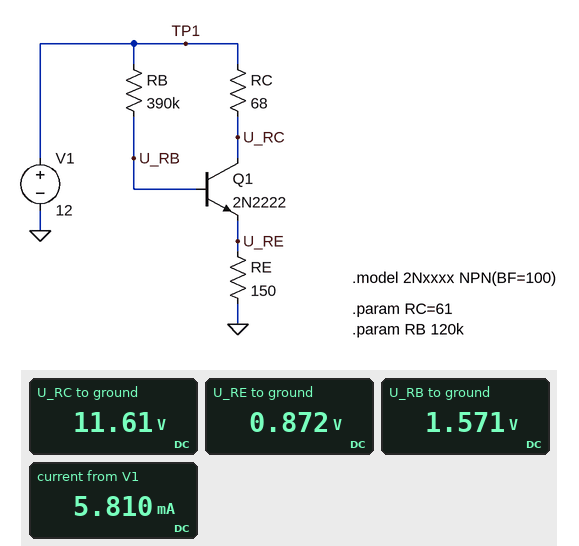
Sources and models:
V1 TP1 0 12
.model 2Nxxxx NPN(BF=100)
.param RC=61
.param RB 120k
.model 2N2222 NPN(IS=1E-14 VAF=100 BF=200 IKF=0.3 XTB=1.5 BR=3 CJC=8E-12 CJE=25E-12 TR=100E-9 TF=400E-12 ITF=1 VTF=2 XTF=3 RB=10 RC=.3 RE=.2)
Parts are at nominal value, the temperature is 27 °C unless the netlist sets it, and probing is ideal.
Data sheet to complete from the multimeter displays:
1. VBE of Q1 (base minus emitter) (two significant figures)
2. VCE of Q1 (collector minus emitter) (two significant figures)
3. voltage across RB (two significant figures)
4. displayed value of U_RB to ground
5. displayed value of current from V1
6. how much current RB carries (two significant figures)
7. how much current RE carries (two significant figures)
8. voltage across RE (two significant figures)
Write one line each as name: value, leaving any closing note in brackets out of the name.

VBE of Q1 (base minus emitter): 700 mV
VCE of Q1 (collector minus emitter): 11 V
voltage across RB: 10 V
displayed value of U_RB to ground: 1.571 V
displayed value of current from V1: 5.810 mA
how much current RB carries: 27 µA
how much current RE carries: 5.8 mA
voltage across RE: 870 mV
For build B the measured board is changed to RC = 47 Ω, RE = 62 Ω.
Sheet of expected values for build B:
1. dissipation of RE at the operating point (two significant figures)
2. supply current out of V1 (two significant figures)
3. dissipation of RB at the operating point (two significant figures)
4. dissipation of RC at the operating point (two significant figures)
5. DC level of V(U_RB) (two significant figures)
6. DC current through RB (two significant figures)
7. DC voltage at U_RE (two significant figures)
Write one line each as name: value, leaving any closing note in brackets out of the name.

dissipation of RE at the operating point: 2.3 mW
supply current out of V1: 6.1 mA
dissipation of RB at the operating point: 310 µW
dissipation of RC at the operating point: 1.7 mW
DC level of V(U_RB): 1.1 V
DC current through RB: 28 µA
DC voltage at U_RE: 380 mV
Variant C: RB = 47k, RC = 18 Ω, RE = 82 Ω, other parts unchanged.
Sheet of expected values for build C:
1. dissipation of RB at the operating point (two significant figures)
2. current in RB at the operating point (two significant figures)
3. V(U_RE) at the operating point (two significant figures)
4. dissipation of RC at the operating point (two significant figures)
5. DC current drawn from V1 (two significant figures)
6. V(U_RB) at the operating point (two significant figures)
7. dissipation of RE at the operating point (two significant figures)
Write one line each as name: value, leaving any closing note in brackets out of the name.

dissipation of RB at the operating point: 1.5 mW
current in RB at the operating point: 180 µA
V(U_RE) at the operating point: 2.9 V
dissipation of RC at the operating point: 22 mW
DC current drawn from V1: 35 mA
V(U_RB) at the operating point: 3.6 V
dissipation of RE at the operating point: 100 mW
